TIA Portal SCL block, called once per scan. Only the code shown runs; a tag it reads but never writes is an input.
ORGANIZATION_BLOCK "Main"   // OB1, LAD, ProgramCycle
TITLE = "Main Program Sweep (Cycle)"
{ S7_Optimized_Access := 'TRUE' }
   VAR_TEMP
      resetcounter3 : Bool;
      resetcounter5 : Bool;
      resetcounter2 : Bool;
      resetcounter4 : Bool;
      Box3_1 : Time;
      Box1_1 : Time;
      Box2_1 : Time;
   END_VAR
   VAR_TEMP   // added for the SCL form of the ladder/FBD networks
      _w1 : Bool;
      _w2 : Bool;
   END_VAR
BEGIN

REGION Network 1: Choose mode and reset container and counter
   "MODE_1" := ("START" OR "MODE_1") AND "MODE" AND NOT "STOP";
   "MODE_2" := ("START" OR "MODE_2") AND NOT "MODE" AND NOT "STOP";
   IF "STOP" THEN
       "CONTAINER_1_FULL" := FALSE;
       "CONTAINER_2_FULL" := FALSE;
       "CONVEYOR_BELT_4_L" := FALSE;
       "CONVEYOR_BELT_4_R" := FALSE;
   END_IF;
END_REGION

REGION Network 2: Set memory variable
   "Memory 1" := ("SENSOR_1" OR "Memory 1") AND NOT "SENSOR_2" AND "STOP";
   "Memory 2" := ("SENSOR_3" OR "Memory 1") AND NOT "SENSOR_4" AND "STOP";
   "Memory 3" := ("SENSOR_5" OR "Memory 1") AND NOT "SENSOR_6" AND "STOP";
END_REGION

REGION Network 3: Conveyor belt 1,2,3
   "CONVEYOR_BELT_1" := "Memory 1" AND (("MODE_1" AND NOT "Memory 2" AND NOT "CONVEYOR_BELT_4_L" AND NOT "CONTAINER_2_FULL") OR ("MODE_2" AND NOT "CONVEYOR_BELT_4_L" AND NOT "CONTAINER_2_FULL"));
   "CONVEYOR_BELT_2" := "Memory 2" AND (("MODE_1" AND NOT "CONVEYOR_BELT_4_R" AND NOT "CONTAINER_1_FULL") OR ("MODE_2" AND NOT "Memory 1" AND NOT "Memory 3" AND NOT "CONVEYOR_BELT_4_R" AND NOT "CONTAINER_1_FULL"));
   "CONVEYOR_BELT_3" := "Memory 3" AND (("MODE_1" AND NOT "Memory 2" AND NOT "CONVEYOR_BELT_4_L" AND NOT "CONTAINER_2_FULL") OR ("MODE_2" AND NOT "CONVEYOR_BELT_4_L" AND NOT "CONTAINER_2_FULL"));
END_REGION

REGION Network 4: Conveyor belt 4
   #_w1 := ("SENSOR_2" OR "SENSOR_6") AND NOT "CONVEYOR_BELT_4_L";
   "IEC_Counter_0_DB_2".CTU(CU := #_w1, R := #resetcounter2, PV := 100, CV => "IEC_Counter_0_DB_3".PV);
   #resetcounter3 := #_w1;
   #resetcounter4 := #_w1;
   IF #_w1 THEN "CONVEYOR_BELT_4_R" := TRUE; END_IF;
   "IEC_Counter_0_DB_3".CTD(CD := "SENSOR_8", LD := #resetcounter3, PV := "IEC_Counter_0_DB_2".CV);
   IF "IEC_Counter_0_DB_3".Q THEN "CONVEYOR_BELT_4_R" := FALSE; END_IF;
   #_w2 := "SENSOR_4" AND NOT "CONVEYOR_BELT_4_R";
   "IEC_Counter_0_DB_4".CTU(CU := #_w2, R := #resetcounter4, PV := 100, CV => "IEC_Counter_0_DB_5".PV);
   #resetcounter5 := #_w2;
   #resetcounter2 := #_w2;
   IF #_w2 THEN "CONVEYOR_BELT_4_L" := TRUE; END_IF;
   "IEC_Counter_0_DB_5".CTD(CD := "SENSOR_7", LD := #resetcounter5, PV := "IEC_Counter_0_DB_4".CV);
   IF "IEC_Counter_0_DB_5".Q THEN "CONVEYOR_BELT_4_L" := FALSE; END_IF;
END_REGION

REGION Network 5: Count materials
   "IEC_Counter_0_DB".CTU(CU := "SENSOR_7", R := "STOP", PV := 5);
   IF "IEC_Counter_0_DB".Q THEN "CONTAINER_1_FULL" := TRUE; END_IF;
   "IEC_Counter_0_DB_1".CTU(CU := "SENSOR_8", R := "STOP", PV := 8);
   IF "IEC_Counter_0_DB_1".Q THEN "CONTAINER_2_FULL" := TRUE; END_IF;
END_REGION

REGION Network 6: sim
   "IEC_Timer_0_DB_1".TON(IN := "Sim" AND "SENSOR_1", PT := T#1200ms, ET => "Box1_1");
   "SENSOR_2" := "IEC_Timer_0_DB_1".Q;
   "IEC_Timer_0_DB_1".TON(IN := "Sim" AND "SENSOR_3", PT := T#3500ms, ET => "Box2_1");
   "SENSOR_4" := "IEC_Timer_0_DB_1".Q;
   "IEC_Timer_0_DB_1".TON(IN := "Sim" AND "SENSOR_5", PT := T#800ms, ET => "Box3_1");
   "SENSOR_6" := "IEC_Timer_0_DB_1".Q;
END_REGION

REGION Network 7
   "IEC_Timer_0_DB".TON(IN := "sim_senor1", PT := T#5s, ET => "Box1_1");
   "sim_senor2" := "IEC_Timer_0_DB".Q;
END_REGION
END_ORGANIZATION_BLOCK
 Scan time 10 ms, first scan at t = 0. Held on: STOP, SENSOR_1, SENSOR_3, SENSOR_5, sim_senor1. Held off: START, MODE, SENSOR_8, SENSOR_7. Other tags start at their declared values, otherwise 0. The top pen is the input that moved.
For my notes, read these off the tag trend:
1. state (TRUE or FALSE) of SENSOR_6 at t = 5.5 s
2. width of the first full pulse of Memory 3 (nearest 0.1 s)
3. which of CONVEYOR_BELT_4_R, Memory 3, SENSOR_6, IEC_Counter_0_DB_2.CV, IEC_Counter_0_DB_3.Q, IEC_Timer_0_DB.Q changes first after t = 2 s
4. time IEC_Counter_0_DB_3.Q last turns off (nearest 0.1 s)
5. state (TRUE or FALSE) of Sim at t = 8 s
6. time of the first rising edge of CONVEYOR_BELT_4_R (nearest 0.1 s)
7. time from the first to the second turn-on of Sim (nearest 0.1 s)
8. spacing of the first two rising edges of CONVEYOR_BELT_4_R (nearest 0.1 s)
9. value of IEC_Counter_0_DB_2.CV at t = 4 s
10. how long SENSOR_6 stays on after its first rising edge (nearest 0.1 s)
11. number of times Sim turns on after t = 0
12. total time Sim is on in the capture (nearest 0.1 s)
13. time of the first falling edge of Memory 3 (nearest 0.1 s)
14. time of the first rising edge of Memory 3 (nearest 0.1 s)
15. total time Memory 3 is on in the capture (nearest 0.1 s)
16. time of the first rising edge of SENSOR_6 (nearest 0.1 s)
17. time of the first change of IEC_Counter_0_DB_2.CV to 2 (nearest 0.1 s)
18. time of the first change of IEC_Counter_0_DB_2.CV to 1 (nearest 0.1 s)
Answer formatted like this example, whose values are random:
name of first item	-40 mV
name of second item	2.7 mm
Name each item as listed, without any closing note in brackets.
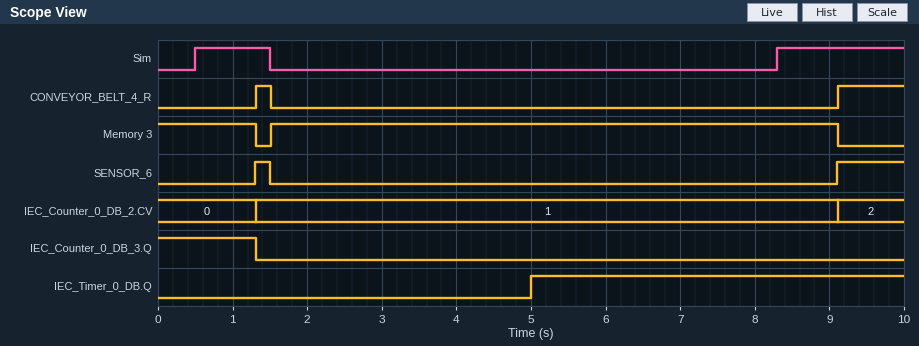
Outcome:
state (TRUE or FALSE) of SENSOR_6 at t = 5.5 s	FALSE
width of the first full pulse of Memory 3	7.6 s
which of CONVEYOR_BELT_4_R, Memory 3, SENSOR_6, IEC_Counter_0_DB_2.CV, IEC_Counter_0_DB_3.Q, IEC_Timer_0_DB.Q changes first after t = 2 s	IEC_Timer_0_DB.Q
time IEC_Counter_0_DB_3.Q last turns off	1.3 s
state (TRUE or FALSE) of Sim at t = 8 s	FALSE
time of the first rising edge of CONVEYOR_BELT_4_R	1.3 s
time from the first to the second turn-on of Sim	7.8 s
spacing of the first two rising edges of CONVEYOR_BELT_4_R	7.8 s
value of IEC_Counter_0_DB_2.CV at t = 4 s	1
how long SENSOR_6 stays on after its first rising edge	0.2 s
number of times Sim turns on after t = 0	2
total time Sim is on in the capture	2.7 s
time of the first falling edge of Memory 3	1.3 s
time of the first rising edge of Memory 3	1.5 s
total time Memory 3 is on in the capture	8.9 s
time of the first rising edge of SENSOR_6	1.3 s
time of the first change of IEC_Counter_0_DB_2.CV to 2	9.1 s
time of the first change of IEC_Counter_0_DB_2.CV to 1	1.3 s
